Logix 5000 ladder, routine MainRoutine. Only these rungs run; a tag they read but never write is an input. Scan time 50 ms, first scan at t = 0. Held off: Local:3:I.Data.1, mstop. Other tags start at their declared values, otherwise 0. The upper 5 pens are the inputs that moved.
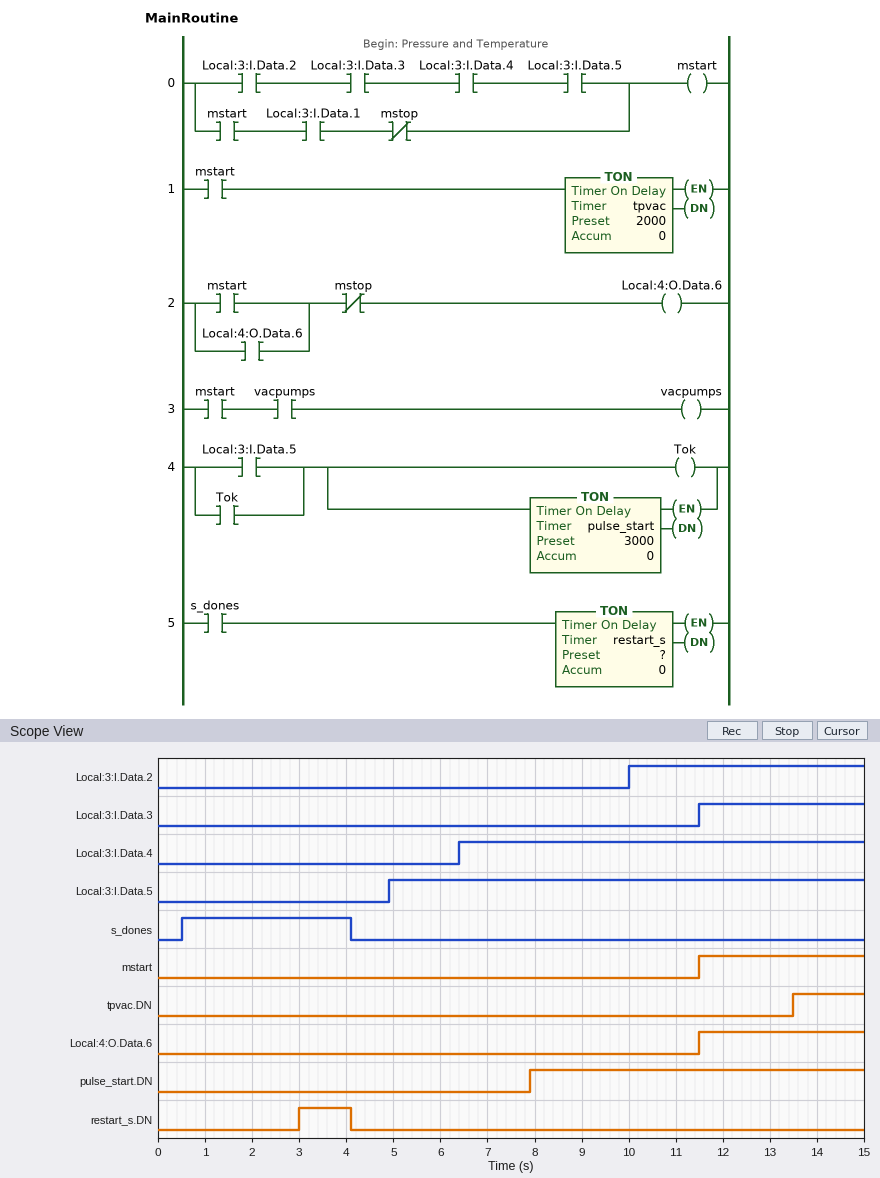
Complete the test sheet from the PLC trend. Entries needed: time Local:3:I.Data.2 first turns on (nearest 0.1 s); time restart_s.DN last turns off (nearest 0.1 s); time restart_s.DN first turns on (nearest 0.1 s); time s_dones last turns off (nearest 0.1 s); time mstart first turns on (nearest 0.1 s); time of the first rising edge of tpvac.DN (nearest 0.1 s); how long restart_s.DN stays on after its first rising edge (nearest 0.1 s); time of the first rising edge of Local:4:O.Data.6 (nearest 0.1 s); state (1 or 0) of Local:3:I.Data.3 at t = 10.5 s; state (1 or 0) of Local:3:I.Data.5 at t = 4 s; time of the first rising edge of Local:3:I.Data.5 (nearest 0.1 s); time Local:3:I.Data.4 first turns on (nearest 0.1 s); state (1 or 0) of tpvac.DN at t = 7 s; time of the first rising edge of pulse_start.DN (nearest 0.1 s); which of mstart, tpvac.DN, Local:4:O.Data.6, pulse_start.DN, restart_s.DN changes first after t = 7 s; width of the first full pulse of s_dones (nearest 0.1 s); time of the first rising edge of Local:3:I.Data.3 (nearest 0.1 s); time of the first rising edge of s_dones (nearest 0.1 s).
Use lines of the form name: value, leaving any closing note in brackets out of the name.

time Local:3:I.Data.2 first turns on: 10.0 s
time restart_s.DN last turns off: 4.1 s
time restart_s.DN first turns on: 3.0 s
time s_dones last turns off: 4.1 s
time mstart first turns on: 11.5 s
time of the first rising edge of tpvac.DN: 13.5 s
how long restart_s.DN stays on after its first rising edge: 1.1 s
time of the first rising edge of Local:4:O.Data.6: 11.5 s
state (1 or 0) of Local:3:I.Data.3 at t = 10.5 s: 0
state (1 or 0) of Local:3:I.Data.5 at t = 4 s: 0
time of the first rising edge of Local:3:I.Data.5: 4.9 s
time Local:3:I.Data.4 first turns on: 6.4 s
state (1 or 0) of tpvac.DN at t = 7 s: 0
time of the first rising edge of pulse_start.DN: 7.9 s
which of mstart, tpvac.DN, Local:4:O.Data.6, pulse_start.DN, restart_s.DN changes first after t = 7 s: pulse_start.DN
width of the first full pulse of s_dones: 3.6 s
time of the first rising edge of Local:3:I.Data.3: 11.5 s
time of the first rising edge of s_dones: 0.5 s
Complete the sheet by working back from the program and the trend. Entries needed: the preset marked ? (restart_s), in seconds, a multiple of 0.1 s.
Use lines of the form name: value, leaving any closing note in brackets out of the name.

the preset marked ? (restart_s), in seconds, a multiple of 0.1 s: 2.5 s
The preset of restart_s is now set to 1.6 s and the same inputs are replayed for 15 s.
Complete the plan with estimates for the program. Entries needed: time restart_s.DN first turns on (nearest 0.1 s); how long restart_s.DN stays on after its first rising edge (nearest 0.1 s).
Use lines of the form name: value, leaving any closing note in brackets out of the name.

time restart_s.DN first turns on: 2.1 s
how long restart_s.DN stays on after its first rising edge: 2.0 s
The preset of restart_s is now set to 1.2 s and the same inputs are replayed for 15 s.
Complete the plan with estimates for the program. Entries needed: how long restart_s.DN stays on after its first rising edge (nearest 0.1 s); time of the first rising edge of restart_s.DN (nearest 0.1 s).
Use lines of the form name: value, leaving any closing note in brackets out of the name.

how long restart_s.DN stays on after its first rising edge: 2.4 s
time of the first rising edge of restart_s.DN: 1.7 s
